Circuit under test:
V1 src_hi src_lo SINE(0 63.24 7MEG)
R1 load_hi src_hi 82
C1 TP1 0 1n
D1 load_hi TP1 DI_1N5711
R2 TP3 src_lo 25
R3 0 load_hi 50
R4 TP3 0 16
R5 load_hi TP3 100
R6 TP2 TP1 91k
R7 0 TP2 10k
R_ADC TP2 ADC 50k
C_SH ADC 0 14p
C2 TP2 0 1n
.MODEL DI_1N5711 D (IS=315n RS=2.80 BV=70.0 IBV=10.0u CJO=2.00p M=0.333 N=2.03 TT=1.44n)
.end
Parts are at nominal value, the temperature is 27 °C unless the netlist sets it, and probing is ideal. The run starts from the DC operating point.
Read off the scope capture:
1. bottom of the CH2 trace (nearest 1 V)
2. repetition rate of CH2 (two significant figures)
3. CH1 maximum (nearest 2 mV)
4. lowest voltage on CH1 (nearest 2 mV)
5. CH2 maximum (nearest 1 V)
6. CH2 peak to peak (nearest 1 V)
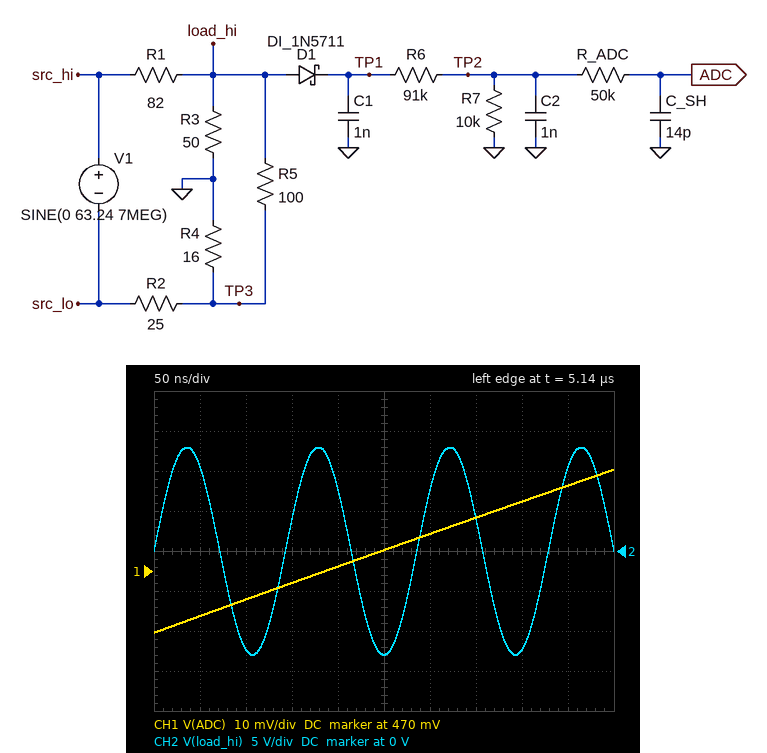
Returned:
-13 V
7.0 MHz
496 mV
454 mV
13 V
26 V
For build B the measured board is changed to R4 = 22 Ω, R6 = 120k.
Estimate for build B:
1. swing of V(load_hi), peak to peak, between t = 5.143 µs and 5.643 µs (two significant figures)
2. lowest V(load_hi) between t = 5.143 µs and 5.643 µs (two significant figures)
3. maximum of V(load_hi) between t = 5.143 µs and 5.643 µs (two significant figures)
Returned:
25 V
-12 V
12 V
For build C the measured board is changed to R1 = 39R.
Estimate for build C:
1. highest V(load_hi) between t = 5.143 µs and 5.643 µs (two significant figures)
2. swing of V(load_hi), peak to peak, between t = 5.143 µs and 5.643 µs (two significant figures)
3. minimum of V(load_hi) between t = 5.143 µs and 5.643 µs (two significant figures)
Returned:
18 V
37 V
-18 V
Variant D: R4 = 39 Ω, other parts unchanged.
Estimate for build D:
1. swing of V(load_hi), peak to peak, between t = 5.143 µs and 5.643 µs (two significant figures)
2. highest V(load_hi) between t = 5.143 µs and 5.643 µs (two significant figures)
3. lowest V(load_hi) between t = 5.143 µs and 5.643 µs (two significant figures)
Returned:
22 V
11 V
-11 V
